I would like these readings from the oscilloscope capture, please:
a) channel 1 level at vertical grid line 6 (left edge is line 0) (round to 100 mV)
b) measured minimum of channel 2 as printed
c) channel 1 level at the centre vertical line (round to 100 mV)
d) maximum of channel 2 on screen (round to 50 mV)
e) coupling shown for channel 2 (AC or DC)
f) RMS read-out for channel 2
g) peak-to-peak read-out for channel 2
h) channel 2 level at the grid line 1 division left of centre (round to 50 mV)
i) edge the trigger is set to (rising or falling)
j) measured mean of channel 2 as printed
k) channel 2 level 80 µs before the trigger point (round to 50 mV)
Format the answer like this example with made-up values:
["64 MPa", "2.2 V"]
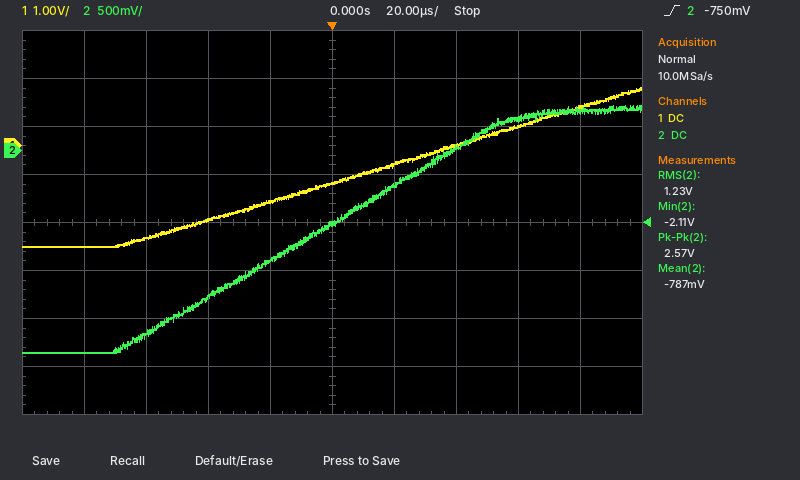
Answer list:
["-400 mV", "-2.11 V", "-800 mV", "450 mV", "DC", "1.23 V", "2.57 V", "-1.15 V", "rising", "-787 mV", "-2.10 V"]
